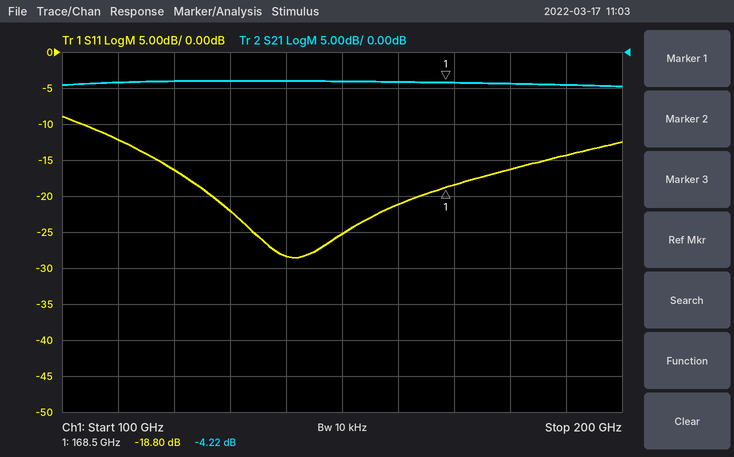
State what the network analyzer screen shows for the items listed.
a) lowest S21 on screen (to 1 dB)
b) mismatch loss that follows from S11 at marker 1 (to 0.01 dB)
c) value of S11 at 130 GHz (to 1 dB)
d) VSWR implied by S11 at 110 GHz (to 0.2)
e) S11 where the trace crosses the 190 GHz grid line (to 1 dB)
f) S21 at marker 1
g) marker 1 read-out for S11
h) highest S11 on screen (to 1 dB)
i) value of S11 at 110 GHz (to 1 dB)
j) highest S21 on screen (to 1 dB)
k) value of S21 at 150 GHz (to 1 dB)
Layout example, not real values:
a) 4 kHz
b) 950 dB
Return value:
a) -5 dB
b) 0.06 dB
c) -22 dB
d) 1.6
e) -14 dB
f) -4.22 dB
g) -18.80 dB
h) -9 dB
i) -12 dB
j) -4 dB
k) -4 dB
